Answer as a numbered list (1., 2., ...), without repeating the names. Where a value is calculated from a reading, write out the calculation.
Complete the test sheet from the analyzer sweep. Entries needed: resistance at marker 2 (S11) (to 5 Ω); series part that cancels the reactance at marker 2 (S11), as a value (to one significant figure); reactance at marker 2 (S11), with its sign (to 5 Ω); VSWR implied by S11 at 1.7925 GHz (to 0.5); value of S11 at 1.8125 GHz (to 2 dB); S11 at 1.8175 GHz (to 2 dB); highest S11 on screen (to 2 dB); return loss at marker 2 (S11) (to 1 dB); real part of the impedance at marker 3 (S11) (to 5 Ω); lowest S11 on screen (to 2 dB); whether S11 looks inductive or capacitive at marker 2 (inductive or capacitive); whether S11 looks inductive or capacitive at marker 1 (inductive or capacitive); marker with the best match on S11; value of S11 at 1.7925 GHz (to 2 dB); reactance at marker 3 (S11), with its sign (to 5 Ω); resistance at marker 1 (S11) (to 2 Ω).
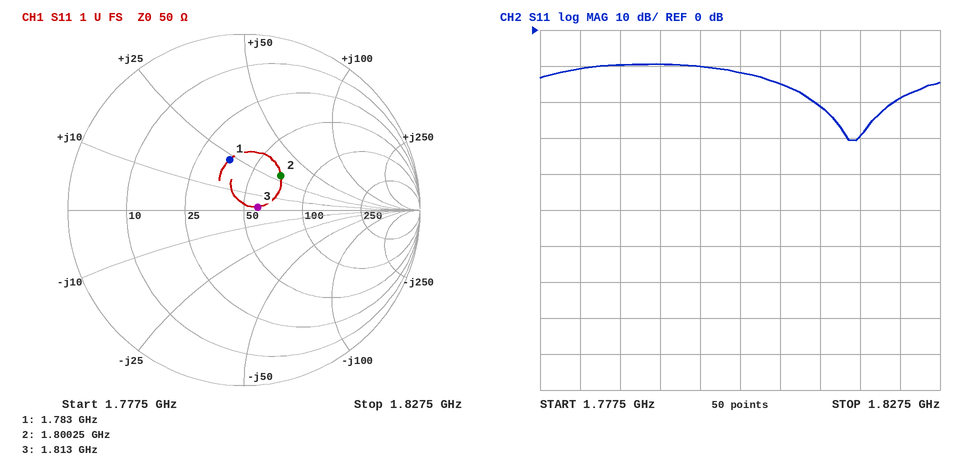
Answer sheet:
1. 70 Ω
2. C = 1/(2π × 1.80025 GHz × 30 Ω) ≈ 3 pF
3. +30 Ω
4. |Γ| = 10^(-10/20) = 0.3162; VSWR = (1 + 0.3162)/(1 − 0.3162) ≈ 1.92, so 2.0 to the nearest 0.5
5. -22 dB
6. -30 dB
7. -10 dB
8. 11 dB
9. 60 Ω
10. -30 dB
11. inductive
12. inductive
13. marker 3
14. -10 dB
15. 0 Ω
16. 36 Ω
